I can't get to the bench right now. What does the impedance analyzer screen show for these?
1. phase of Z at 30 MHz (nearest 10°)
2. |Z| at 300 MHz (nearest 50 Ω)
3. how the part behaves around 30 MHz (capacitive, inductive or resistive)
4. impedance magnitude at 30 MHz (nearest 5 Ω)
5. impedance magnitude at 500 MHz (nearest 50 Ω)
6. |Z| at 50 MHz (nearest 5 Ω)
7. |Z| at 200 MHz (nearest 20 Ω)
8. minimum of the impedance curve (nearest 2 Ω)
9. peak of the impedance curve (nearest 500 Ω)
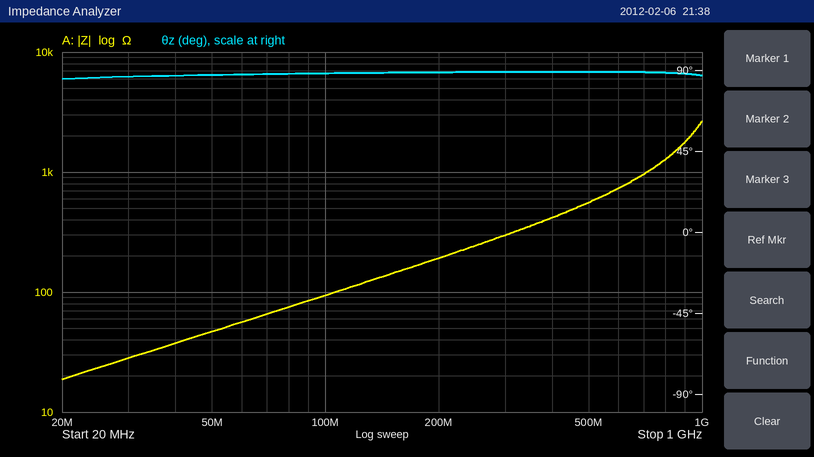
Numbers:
90°
300 Ω
inductive
30 Ω
550 Ω
45 Ω
200 Ω
18 Ω
2.5 kΩ
